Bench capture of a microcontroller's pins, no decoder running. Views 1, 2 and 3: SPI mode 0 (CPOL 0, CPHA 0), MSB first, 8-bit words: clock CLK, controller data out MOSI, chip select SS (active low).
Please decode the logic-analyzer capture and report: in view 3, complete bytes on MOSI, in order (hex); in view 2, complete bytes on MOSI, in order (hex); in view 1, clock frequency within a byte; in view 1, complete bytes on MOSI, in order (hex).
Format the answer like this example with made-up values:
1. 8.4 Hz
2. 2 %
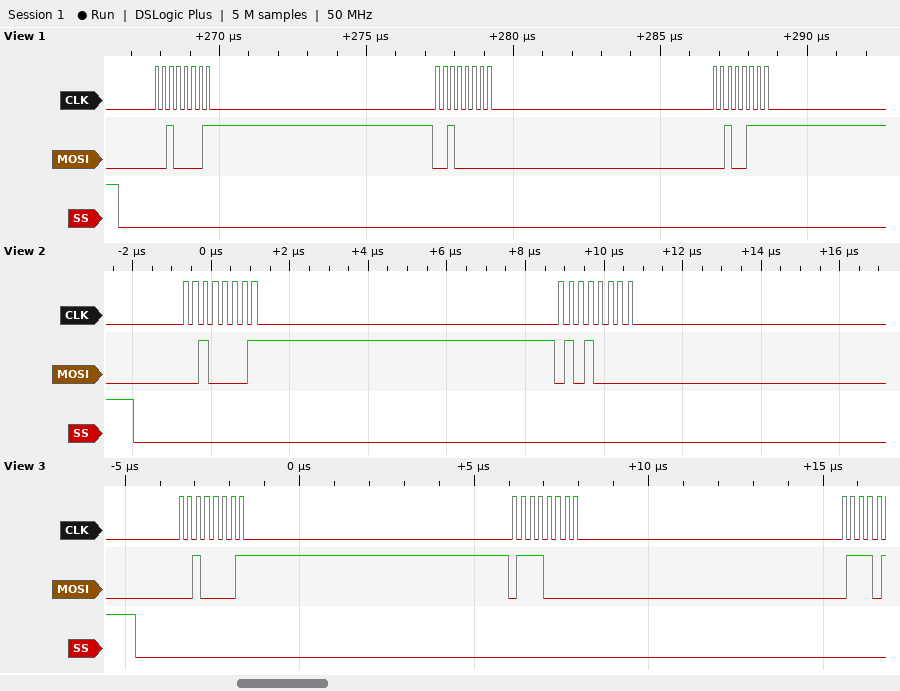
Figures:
1. 21 70
2. 0x21 0x50
3. 4 MHz
4. 0x21 0x20 0x27
